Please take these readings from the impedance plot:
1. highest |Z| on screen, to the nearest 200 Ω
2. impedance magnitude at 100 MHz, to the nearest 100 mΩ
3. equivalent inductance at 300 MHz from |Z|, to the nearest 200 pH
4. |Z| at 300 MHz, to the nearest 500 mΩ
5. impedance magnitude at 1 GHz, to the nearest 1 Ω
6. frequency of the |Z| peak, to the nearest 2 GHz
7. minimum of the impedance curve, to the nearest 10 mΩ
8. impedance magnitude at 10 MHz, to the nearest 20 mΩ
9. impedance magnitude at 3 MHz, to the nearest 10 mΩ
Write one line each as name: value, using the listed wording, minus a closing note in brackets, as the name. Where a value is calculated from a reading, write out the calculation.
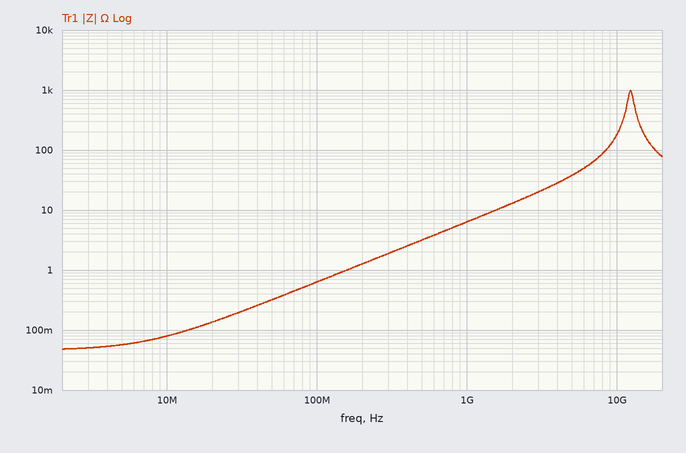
highest |Z| on screen, to the nearest 200 Ω: 1.0 kΩ
impedance magnitude at 100 MHz, to the nearest 100 mΩ: 600 mΩ
equivalent inductance at 300 MHz from |Z|, to the nearest 200 pH: L = 2.0 Ω/(2π × 300 MHz) ≈ 1.06 nH, so 1.0 nH to the nearest 200 pH
|Z| at 300 MHz, to the nearest 500 mΩ: 2.0 Ω
impedance magnitude at 1 GHz, to the nearest 1 Ω: 6 Ω
frequency of the |Z| peak, to the nearest 2 GHz: 12 GHz
minimum of the impedance curve, to the nearest 10 mΩ: 50 mΩ
impedance magnitude at 10 MHz, to the nearest 20 mΩ: 80 mΩ
impedance magnitude at 3 MHz, to the nearest 10 mΩ: 50 mΩ
